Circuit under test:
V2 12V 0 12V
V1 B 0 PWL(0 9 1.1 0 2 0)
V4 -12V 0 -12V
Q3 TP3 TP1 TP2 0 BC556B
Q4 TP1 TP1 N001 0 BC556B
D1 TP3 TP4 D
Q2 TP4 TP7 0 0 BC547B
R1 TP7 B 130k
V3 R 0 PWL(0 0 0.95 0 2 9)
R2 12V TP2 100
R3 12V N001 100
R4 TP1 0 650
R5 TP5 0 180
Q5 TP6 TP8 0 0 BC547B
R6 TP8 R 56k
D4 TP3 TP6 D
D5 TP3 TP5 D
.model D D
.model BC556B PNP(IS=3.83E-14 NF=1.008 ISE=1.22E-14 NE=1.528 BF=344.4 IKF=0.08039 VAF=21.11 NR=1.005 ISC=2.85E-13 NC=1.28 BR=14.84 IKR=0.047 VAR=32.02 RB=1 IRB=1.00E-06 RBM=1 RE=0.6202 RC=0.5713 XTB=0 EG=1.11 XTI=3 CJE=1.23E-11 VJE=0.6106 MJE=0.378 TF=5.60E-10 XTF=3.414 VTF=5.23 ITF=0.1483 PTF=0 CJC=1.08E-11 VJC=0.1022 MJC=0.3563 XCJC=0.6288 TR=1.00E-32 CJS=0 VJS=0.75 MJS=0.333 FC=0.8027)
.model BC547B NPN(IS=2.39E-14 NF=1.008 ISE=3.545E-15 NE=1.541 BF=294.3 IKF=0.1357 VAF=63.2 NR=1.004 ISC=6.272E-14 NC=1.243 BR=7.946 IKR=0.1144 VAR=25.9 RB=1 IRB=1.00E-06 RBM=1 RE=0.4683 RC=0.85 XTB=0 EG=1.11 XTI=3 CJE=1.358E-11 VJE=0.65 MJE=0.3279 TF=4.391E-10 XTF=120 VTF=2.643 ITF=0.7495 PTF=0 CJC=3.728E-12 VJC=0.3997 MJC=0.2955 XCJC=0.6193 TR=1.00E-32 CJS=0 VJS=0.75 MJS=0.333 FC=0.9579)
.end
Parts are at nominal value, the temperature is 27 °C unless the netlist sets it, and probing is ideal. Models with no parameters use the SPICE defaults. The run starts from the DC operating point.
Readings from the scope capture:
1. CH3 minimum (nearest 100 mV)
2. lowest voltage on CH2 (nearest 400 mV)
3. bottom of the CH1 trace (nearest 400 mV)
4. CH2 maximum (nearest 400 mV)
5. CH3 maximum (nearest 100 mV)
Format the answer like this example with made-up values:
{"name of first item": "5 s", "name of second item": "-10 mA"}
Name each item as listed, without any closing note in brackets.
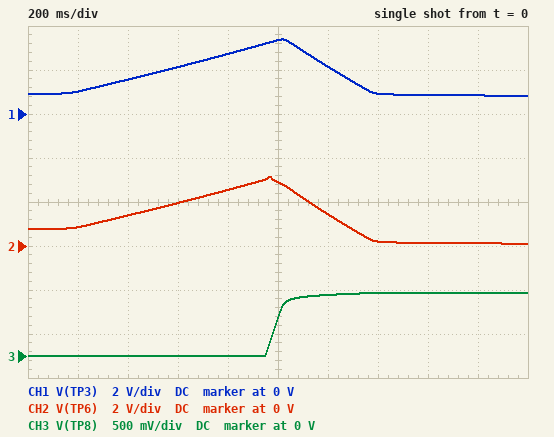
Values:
{"CH3 minimum": "0 V", "lowest voltage on CH2": "0 V", "bottom of the CH1 trace": "800 mV", "CH2 maximum": "3.2 V", "CH3 maximum": "700 mV"}
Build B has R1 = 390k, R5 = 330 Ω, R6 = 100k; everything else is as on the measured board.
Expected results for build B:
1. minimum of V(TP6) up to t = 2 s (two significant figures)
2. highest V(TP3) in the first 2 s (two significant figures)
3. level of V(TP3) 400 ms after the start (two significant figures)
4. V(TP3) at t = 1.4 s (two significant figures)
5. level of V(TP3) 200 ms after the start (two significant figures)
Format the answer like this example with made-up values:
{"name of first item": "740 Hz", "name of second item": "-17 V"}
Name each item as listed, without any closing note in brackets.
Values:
{"minimum of V(TP6) up to t = 2 s": "140 mV", "highest V(TP3) in the first 2 s": "5.6 V", "level of V(TP3) 400 ms after the start": "4.4 V", "V(TP3) at t = 1.4 s": "2.8 V", "level of V(TP3) 200 ms after the start": "4.1 V"}
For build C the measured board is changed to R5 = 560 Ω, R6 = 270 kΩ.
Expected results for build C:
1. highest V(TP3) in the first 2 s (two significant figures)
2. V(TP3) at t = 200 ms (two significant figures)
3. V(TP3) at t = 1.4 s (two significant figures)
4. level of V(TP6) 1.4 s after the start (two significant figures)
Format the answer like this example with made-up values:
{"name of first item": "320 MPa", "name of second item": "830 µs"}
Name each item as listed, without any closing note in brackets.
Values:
{"highest V(TP3) in the first 2 s": "9.0 V", "V(TP3) at t = 200 ms": "1.7 V", "V(TP3) at t = 1.4 s": "7.1 V", "level of V(TP6) 1.4 s after the start": "6.4 V"}
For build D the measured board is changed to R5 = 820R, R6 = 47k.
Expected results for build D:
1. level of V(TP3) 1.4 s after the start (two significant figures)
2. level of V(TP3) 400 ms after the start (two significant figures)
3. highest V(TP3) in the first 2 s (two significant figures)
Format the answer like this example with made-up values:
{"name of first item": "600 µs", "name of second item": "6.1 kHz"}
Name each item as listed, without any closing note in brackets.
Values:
{"level of V(TP3) 1.4 s after the start": "900 mV", "level of V(TP3) 400 ms after the start": "4.3 V", "highest V(TP3) in the first 2 s": "11 V"}
